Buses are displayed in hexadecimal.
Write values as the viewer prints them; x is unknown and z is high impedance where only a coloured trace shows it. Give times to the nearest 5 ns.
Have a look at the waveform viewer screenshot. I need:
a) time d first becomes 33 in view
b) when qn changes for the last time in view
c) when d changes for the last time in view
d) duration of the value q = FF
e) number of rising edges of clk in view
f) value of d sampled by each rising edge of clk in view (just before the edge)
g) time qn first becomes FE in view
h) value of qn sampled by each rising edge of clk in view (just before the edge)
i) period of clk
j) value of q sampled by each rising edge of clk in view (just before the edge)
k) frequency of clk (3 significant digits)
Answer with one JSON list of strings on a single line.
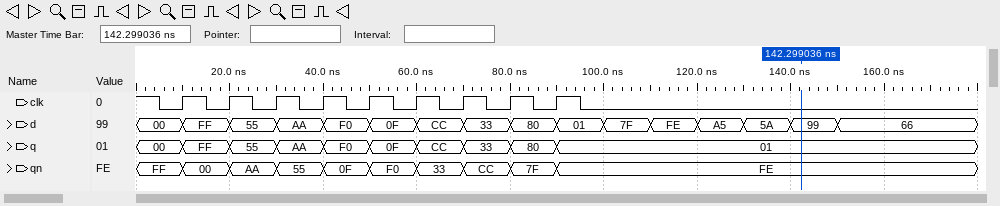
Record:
["70 ns", "90 ns", "150 ns", "10 ns", "9", "00, FF, 55, AA, F0, 0F, CC, 33, 80", "90 ns", "FF, 00, AA, 55, 0F, F0, 33, CC, 7F", "10 ns", "00, FF, 55, AA, F0, 0F, CC, 33, 80", "100 MHz"]
